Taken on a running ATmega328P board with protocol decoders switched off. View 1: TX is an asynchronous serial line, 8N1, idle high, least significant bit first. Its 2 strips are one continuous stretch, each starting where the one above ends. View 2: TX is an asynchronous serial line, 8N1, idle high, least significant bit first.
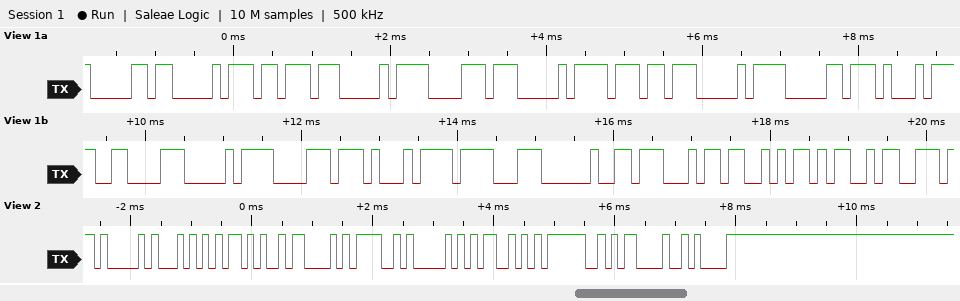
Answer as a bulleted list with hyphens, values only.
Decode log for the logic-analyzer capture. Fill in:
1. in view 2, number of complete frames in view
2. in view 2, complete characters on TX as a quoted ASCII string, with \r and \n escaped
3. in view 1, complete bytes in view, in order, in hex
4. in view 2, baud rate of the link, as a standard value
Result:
- 10
- "AT+COPS?\r\n"
- B0 D0 BB D0 B8 D0 B7 D0 B0 D1 86 D0 B8 D1 8F 20 47 53 4D
- 9600 baud
